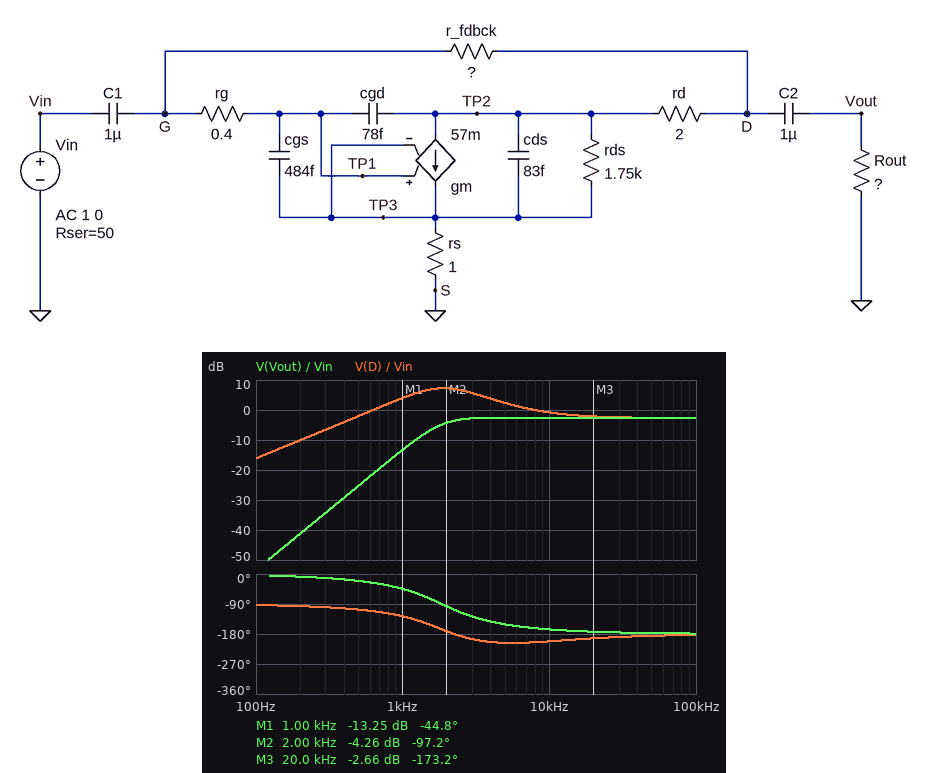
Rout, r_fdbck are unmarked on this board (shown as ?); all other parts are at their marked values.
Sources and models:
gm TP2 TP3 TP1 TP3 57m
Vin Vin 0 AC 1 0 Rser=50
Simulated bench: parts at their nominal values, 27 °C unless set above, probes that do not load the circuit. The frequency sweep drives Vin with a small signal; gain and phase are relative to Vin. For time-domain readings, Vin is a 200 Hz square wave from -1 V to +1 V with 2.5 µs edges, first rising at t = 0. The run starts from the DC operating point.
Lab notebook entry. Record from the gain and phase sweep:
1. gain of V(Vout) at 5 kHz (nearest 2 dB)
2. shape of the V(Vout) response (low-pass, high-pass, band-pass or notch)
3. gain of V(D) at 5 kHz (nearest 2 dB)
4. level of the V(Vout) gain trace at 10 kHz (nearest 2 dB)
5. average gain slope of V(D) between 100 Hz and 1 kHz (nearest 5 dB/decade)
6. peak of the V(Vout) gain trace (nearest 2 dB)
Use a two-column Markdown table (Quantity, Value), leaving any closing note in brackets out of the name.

| Quantity | Value |
|---|---|
| gain of V(Vout) at 5 kHz | -2 dB |
| shape of the V(Vout) response | high-pass |
| gain of V(D) at 5 kHz | 2 dB |
| level of the V(Vout) gain trace at 10 kHz | -2 dB |
| average gain slope of V(D) between 100 Hz and 1 kHz | 20 dB/decade |
| peak of the V(Vout) gain trace | -2 dB |
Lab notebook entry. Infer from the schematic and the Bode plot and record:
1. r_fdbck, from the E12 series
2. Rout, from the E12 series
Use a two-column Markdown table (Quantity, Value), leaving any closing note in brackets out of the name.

| Quantity | Value |
|---|---|
| r_fdbck, from the E12 series | 270 Ω |
| Rout, from the E12 series | 22 Ω |
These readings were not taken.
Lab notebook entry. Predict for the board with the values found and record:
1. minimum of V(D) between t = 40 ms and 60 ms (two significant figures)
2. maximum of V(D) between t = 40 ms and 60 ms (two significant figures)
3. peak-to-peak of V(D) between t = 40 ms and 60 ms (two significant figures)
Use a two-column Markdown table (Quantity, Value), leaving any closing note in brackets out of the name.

| Quantity | Value |
|---|---|
| minimum of V(D) between t = 40 ms and 60 ms | -2.9 V |
| maximum of V(D) between t = 40 ms and 60 ms | 2.9 V |
| peak-to-peak of V(D) between t = 40 ms and 60 ms | 5.8 V |
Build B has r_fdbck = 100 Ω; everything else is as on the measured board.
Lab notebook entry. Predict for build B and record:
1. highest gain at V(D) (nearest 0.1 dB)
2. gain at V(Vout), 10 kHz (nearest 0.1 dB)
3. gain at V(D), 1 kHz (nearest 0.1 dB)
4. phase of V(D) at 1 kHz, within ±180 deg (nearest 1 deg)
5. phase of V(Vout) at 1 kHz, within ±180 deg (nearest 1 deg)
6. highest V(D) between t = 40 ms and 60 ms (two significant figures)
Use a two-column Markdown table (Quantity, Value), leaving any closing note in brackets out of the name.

| Quantity | Value |
|---|---|
| highest gain at V(D) | -2.2 dB |
| gain at V(Vout), 10 kHz | -7.9 dB |
| gain at V(D), 1 kHz | -6.5 dB |
| phase of V(D) at 1 kHz, within ±180 deg | -122 deg |
| phase of V(Vout) at 1 kHz, within ±180 deg | -40 deg |
| highest V(D) between t = 40 ms and 60 ms | 1.1 V |
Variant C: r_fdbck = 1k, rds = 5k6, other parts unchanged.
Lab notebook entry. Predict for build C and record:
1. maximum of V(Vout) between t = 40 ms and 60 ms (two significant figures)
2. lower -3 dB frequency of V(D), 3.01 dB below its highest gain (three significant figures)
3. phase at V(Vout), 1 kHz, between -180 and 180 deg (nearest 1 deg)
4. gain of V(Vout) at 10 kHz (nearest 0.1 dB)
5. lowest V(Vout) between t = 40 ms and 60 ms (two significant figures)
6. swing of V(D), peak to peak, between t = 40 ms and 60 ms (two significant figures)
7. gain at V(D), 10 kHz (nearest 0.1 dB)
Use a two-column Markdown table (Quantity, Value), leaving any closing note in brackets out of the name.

| Quantity | Value |
|---|---|
| maximum of V(Vout) between t = 40 ms and 60 ms | 2.0 V |
| lower -3 dB frequency of V(D), 3.01 dB below its highest gain | 756 Hz |
| phase at V(Vout), 1 kHz, between -180 and 180 deg | -76 deg |
| gain of V(Vout) at 10 kHz | 0.3 dB |
| lowest V(Vout) between t = 40 ms and 60 ms | -2.0 V |
| swing of V(D), peak to peak, between t = 40 ms and 60 ms | 17 V |
| gain at V(D), 10 kHz | 2.1 dB |
